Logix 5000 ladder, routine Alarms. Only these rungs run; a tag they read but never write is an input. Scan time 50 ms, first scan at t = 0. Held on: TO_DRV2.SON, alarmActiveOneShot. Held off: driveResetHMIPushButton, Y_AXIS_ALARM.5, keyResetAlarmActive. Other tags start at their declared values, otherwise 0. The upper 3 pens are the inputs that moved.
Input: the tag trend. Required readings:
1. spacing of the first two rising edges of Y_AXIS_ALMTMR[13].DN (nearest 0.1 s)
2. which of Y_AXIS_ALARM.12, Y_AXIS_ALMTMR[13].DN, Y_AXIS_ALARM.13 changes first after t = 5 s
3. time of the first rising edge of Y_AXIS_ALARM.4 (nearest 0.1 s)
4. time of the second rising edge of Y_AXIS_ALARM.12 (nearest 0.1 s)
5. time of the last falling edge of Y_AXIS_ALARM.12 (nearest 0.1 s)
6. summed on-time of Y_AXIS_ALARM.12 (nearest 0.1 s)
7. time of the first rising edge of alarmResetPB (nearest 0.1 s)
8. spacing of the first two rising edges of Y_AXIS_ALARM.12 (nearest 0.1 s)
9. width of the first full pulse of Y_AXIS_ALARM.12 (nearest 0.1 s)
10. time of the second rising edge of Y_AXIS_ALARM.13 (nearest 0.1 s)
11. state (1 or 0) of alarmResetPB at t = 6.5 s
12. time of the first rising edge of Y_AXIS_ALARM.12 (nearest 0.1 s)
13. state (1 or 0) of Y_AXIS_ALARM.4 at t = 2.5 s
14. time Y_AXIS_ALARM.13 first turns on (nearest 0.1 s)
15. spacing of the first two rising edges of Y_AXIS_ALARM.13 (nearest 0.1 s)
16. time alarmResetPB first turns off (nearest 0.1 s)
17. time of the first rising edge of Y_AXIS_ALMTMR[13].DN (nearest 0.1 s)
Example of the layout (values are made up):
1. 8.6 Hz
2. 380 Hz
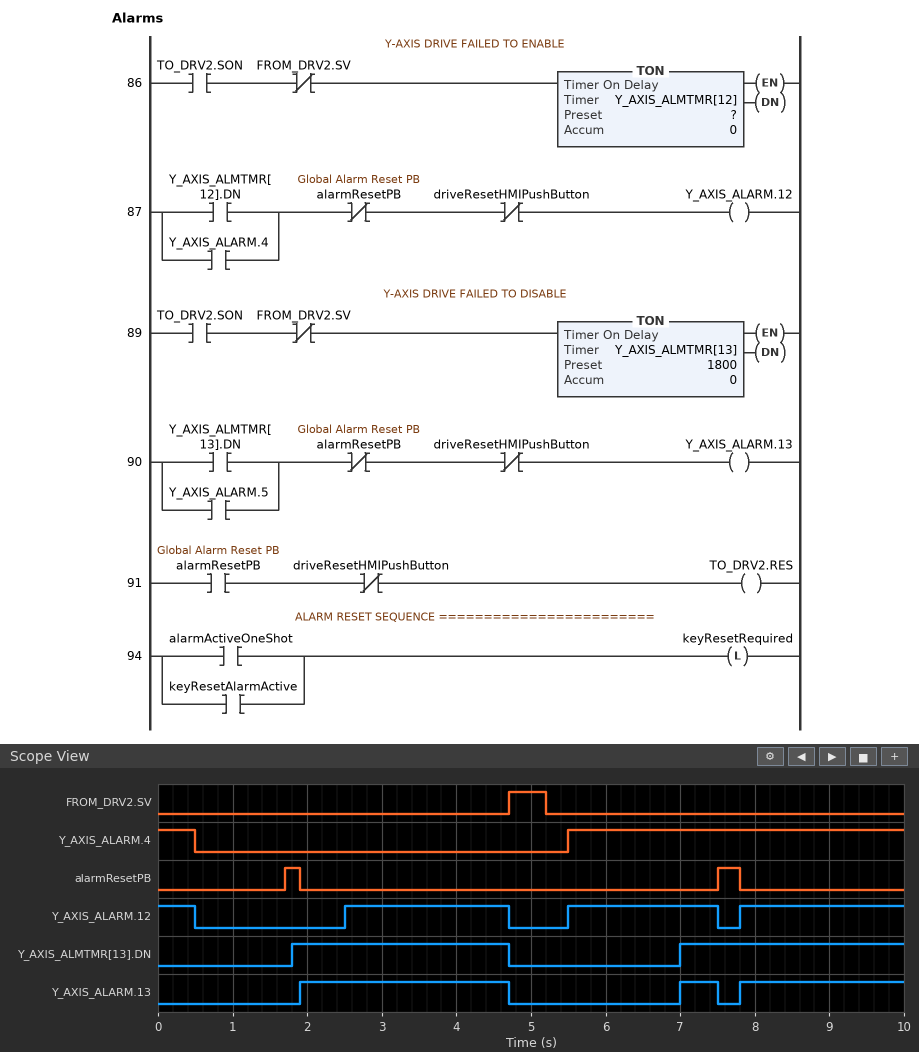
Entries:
1. 5.2 s
2. Y_AXIS_ALARM.12
3. 5.5 s
4. 5.5 s
5. 7.5 s
6. 6.9 s
7. 1.7 s
8. 3.0 s
9. 2.2 s
10. 7.0 s
11. 0
12. 2.5 s
13. 0
14. 1.9 s
15. 5.1 s
16. 1.9 s
17. 1.8 s
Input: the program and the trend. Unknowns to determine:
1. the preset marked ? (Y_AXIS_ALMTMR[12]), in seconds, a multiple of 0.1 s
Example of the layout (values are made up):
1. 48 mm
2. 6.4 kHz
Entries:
1. 2.5 s
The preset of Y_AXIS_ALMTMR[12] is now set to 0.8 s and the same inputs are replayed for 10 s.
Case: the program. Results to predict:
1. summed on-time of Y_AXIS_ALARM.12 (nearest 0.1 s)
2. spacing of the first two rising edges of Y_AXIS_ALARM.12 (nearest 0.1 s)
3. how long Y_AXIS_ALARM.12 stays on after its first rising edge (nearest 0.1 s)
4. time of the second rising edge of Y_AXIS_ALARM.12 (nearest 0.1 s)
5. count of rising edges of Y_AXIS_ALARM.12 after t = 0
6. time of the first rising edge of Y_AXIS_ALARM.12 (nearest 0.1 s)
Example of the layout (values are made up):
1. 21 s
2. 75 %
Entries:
1. 8.4 s
2. 1.1 s
3. 0.9 s
4. 1.9 s
5. 4
6. 0.8 s
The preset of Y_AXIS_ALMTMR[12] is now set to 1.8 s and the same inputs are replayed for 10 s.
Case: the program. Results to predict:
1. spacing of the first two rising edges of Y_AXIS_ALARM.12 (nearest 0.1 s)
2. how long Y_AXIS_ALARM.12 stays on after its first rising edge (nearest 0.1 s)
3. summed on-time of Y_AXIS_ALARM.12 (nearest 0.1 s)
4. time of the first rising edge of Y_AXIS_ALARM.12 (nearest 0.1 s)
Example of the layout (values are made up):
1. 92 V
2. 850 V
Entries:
1. 3.6 s
2. 2.8 s
3. 7.5 s
4. 1.9 s
